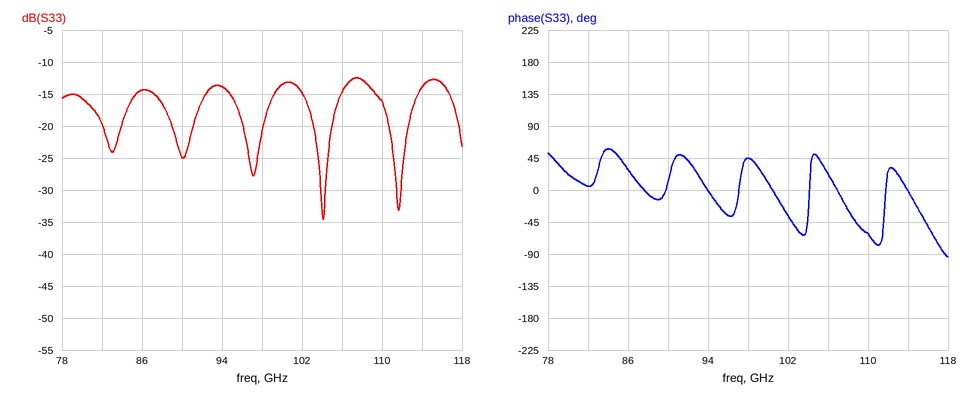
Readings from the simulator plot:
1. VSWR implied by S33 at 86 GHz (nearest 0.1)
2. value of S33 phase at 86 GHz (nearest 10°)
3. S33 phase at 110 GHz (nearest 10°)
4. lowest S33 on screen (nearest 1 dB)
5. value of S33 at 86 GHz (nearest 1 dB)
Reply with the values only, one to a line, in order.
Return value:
1.5
30°
-60°
-35 dB
-14 dB
